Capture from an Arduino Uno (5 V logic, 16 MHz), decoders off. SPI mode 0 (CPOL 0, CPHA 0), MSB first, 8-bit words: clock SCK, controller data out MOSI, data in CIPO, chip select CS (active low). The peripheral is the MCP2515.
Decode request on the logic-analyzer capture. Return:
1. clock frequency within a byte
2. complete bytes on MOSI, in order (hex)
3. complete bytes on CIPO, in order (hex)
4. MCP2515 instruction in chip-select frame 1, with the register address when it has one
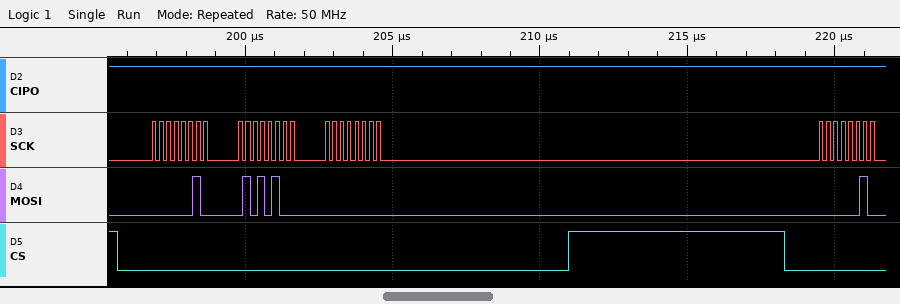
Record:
4 MHz
02 54 00 02
FF FF FF FF
WRITE 0x54
